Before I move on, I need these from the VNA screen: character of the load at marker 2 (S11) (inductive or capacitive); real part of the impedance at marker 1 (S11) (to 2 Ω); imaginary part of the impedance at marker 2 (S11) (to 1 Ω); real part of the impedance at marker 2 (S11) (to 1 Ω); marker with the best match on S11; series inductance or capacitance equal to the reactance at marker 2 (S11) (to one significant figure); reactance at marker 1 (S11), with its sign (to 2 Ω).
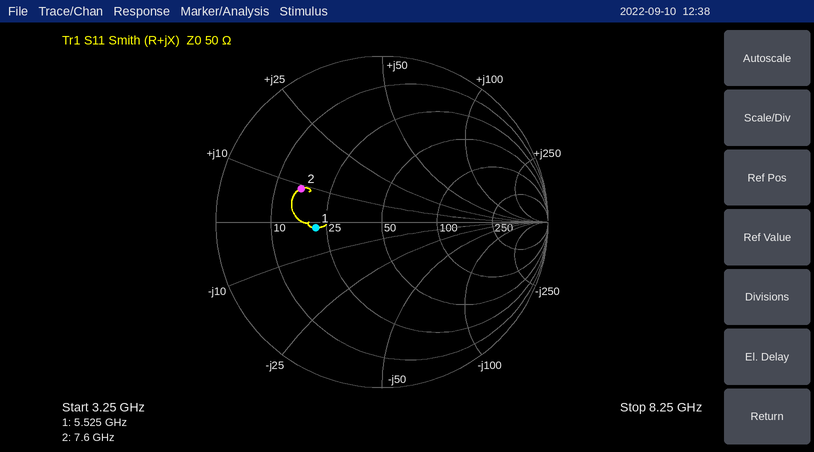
inductive
22 Ω
+9 Ω
16 Ω
marker 1
200 pH
-2 Ω
